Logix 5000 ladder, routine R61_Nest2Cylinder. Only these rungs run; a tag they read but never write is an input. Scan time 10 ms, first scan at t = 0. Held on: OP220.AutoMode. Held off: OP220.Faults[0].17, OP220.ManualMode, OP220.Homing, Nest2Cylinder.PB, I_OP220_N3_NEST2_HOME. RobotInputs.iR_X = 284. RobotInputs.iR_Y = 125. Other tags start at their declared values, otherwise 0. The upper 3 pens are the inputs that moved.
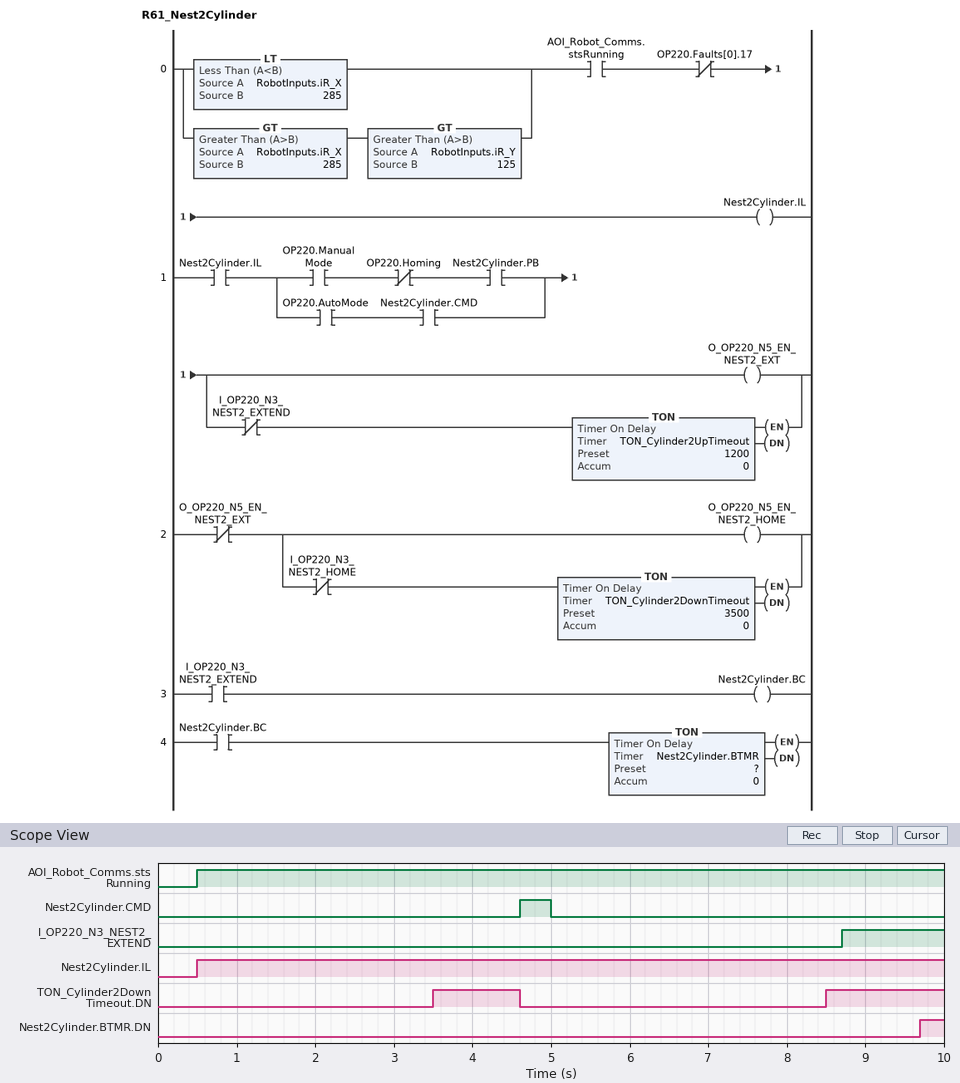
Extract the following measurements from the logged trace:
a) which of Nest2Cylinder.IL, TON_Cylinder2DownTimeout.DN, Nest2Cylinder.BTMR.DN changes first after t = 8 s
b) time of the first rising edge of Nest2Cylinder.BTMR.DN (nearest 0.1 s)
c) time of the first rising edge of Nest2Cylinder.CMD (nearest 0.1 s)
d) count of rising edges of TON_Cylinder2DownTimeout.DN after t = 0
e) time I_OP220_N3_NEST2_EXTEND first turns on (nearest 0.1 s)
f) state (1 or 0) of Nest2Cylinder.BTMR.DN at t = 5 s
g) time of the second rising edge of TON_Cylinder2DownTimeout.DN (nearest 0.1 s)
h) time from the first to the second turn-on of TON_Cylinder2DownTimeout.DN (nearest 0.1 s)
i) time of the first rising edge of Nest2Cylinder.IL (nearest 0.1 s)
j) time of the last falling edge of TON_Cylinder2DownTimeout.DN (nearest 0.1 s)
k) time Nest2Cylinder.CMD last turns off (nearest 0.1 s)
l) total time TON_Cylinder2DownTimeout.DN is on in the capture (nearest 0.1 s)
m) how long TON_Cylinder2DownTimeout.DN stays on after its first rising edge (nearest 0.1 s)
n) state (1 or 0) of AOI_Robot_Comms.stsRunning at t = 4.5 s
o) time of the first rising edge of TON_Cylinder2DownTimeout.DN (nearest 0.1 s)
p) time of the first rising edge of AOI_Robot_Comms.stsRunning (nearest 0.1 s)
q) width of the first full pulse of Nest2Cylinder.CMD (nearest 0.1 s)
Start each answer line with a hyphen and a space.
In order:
- TON_Cylinder2DownTimeout.DN
- 9.7 s
- 4.6 s
- 2
- 8.7 s
- 0
- 8.5 s
- 5.0 s
- 0.5 s
- 4.6 s
- 5.0 s
- 2.6 s
- 1.1 s
- 1
- 3.5 s
- 0.5 s
- 0.4 s
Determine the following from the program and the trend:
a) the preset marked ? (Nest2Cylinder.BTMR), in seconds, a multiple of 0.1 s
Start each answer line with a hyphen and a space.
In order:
- 1.0 s
